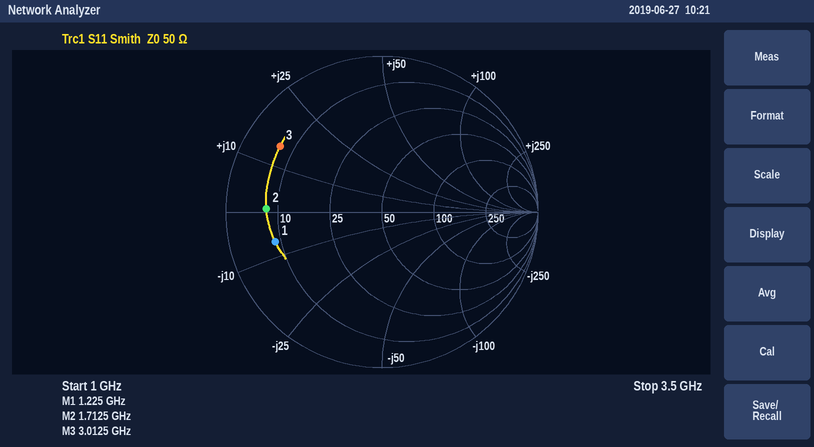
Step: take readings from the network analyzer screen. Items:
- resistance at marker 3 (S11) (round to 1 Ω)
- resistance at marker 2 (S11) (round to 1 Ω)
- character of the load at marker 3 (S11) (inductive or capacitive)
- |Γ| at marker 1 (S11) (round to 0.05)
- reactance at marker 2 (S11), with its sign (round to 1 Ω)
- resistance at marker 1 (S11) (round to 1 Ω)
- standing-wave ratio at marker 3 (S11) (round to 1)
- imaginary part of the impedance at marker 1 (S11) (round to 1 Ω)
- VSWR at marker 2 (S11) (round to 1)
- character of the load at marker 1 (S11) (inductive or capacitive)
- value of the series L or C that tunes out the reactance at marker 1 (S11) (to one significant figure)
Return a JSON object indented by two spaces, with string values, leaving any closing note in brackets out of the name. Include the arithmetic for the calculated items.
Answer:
{
  "resistance at marker 3 (S11)": "7 Ω",
  "resistance at marker 2 (S11)": "7 Ω",
  "character of the load at marker 3 (S11)": "inductive",
  "|Γ| at marker 1 (S11)": "0.70",
  "reactance at marker 2 (S11), with its sign": "+1 Ω",
  "resistance at marker 1 (S11)": "9 Ω",
  "standing-wave ratio at marker 3 (S11)": "8",
  "imaginary part of the impedance at marker 1 (S11)": "-7 Ω",
  "VSWR at marker 2 (S11)": "7",
  "character of the load at marker 1 (S11)": "capacitive",
  "value of the series L or C that tunes out the reactance at marker 1 (S11)": "L = 7 Ω/(2π × 1.225 GHz) ≈ 909 pH, so 900 pH to one significant figure"
}
